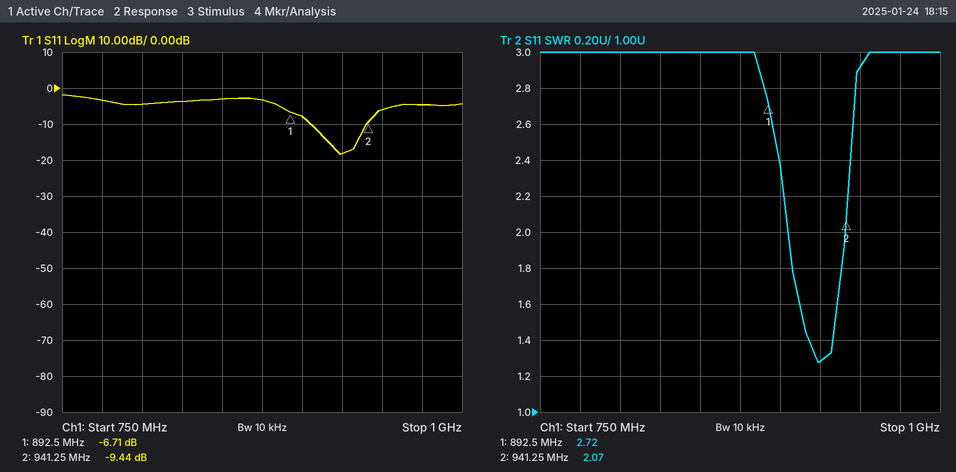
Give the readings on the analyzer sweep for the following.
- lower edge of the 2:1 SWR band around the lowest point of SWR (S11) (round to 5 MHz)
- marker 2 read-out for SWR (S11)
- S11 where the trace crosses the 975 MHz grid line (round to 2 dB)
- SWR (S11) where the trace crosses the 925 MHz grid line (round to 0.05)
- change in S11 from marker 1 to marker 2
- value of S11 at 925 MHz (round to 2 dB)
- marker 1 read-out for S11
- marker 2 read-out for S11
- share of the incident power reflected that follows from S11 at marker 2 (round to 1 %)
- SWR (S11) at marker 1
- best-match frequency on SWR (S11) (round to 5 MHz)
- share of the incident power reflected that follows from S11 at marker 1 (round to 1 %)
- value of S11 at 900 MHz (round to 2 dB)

905 MHz
2.07
-4 dB
1.30
-2.73 dB
-18 dB
-6.71 dB
-9.44 dB
11 %
2.72
925 MHz
21 %
-8 dB
